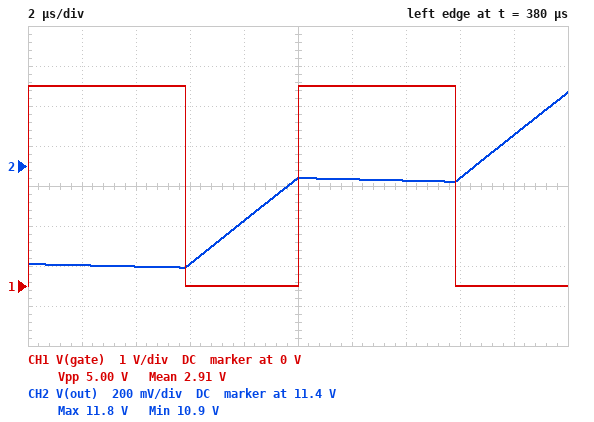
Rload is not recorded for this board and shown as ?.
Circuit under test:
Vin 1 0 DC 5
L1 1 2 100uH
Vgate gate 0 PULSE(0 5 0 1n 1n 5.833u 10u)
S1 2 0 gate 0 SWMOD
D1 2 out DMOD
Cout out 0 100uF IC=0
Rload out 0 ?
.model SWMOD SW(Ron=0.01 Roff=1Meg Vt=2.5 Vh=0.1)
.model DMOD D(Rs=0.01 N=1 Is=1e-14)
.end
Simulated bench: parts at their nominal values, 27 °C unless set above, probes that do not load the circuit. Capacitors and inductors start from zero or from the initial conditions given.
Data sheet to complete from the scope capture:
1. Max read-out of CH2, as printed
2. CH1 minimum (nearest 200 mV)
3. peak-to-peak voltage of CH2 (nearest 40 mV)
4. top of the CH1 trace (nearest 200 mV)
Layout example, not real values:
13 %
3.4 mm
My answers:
11.8 V
0 V
880 mV
5.0 V
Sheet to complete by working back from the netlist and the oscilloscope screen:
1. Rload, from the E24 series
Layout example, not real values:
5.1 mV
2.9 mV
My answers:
36 Ω
